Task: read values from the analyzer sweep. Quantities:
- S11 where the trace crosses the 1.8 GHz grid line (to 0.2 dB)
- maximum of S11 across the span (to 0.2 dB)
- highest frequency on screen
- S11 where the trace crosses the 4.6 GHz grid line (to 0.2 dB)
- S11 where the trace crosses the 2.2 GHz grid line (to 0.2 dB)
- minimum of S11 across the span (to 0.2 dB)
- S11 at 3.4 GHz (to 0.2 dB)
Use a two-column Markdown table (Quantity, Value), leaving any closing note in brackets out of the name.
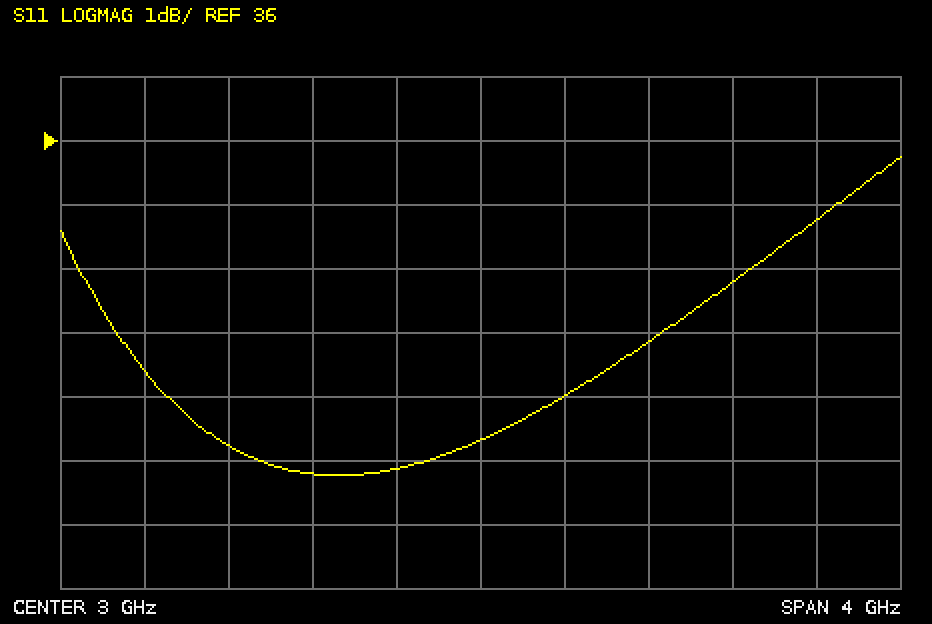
| Quantity | Value |
|---|---|
| S11 where the trace crosses the 1.8 GHz grid line | 31.2 dB |
| maximum of S11 across the span | 35.8 dB |
| highest frequency on screen | 5 GHz |
| S11 where the trace crosses the 4.6 GHz grid line | 34.8 dB |
| S11 where the trace crosses the 2.2 GHz grid line | 30.8 dB |
| minimum of S11 across the span | 30.8 dB |
| S11 at 3.4 GHz | 32.0 dB |
